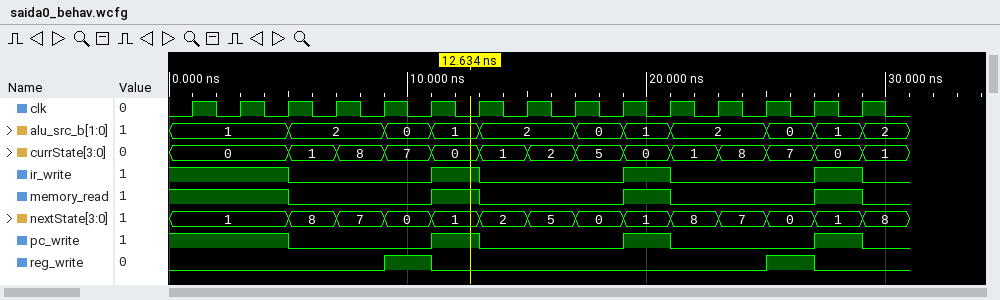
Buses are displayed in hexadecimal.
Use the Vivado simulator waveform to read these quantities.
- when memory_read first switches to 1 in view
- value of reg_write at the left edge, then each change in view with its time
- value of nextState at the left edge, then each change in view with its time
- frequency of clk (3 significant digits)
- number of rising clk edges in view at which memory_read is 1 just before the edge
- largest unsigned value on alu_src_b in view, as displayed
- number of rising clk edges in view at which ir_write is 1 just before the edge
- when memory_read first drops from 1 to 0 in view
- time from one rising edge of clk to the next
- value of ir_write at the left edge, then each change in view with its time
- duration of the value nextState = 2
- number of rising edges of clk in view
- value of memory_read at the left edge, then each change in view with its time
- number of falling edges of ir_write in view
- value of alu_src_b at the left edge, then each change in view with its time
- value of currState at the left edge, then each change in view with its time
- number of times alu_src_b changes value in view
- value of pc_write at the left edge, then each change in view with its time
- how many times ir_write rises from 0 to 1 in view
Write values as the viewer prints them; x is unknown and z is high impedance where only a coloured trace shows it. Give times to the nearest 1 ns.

11 ns
0, 1 at 9 ns, 0 at 11 ns, 1 at 25 ns, 0 at 27 ns
1, 8 at 5 ns, 7 at 7 ns, 0 at 9 ns, 1 at 11 ns, 2 at 13 ns, 5 at 15 ns, 0 at 17 ns, 1 at 19 ns, 8 at 21 ns, 7 at 23 ns, 0 at 25 ns, 1 at 27 ns, 8 at 29 ns
500 MHz
6
2
6
5 ns
2 ns
1, 0 at 5 ns, 1 at 11 ns, 0 at 13 ns, 1 at 19 ns, 0 at 21 ns, 1 at 27 ns, 0 at 29 ns
2 ns
15
1, 0 at 5 ns, 1 at 11 ns, 0 at 13 ns, 1 at 19 ns, 0 at 21 ns, 1 at 27 ns, 0 at 29 ns
4
1, 2 at 5 ns, 0 at 9 ns, 1 at 11 ns, 2 at 13 ns, 0 at 17 ns, 1 at 19 ns, 2 at 21 ns, 0 at 25 ns, 1 at 27 ns, 2 at 29 ns
0, 1 at 5 ns, 8 at 7 ns, 7 at 9 ns, 0 at 11 ns, 1 at 13 ns, 2 at 15 ns, 5 at 17 ns, 0 at 19 ns, 1 at 21 ns, 8 at 23 ns, 7 at 25 ns, 0 at 27 ns, 1 at 29 ns
10
1, 0 at 5 ns, 1 at 11 ns, 0 at 13 ns, 1 at 19 ns, 0 at 21 ns, 1 at 27 ns, 0 at 29 ns
3
